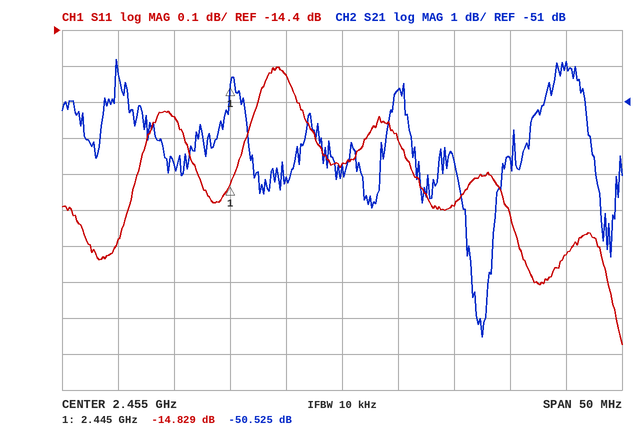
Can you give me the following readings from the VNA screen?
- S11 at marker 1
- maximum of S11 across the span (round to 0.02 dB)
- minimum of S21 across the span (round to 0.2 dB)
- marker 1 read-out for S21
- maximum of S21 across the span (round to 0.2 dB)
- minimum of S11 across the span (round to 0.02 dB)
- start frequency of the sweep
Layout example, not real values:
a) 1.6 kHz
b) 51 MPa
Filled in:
a) -14.829 dB
b) -14.50 dB
c) -57.6 dB
d) -50.525 dB
e) -49.8 dB
f) -15.28 dB
g) 2.43 GHz
